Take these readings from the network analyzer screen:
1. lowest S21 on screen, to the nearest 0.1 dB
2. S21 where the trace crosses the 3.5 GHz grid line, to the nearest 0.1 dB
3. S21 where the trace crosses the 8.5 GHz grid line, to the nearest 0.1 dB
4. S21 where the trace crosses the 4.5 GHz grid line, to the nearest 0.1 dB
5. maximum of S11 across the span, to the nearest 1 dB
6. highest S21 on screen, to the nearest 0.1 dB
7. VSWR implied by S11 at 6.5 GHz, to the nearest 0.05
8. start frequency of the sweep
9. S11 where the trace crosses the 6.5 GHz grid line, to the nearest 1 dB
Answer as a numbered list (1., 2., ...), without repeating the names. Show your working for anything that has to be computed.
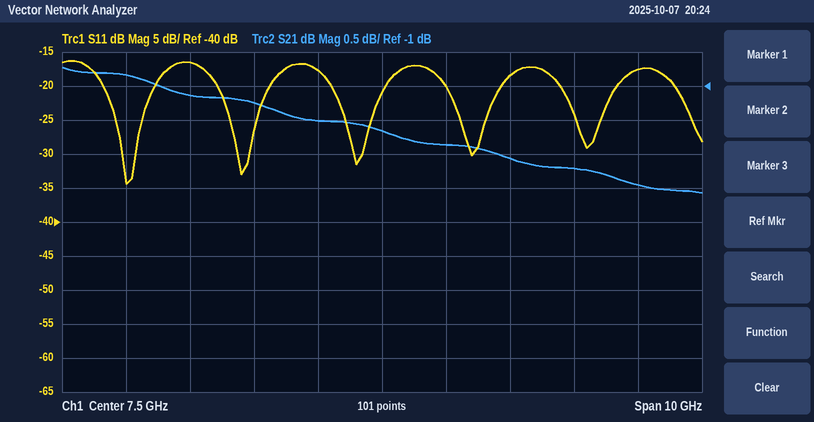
1. -2.6 dB
2. -0.8 dB
3. -1.9 dB
4. -1.1 dB
5. -16 dB
6. -0.7 dB
7. |Γ| = 10^(-18/20) = 0.1259; VSWR = (1 + 0.1259)/(1 − 0.1259) ≈ 1.29, so 1.30 to the nearest 0.05
8. 2.5 GHz
9. -18 dB
